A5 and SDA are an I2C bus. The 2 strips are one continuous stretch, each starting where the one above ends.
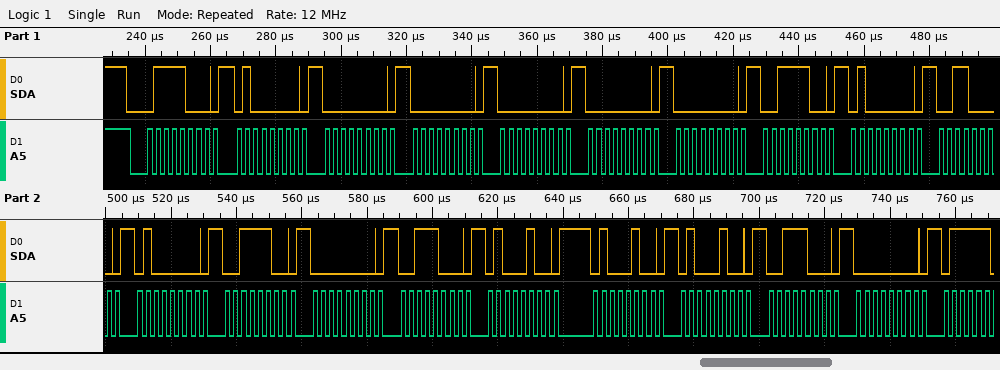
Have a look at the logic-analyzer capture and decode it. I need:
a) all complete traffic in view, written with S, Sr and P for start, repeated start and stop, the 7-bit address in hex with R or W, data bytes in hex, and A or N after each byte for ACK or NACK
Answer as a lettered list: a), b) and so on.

a) S 3CW A 40 A 00 A 00 A 00 A 00 A 00 A 3C A 40 A 30 A 40 A 3C A 00 A 38 A 44 A 44 A 44 A 38 A 00 A
